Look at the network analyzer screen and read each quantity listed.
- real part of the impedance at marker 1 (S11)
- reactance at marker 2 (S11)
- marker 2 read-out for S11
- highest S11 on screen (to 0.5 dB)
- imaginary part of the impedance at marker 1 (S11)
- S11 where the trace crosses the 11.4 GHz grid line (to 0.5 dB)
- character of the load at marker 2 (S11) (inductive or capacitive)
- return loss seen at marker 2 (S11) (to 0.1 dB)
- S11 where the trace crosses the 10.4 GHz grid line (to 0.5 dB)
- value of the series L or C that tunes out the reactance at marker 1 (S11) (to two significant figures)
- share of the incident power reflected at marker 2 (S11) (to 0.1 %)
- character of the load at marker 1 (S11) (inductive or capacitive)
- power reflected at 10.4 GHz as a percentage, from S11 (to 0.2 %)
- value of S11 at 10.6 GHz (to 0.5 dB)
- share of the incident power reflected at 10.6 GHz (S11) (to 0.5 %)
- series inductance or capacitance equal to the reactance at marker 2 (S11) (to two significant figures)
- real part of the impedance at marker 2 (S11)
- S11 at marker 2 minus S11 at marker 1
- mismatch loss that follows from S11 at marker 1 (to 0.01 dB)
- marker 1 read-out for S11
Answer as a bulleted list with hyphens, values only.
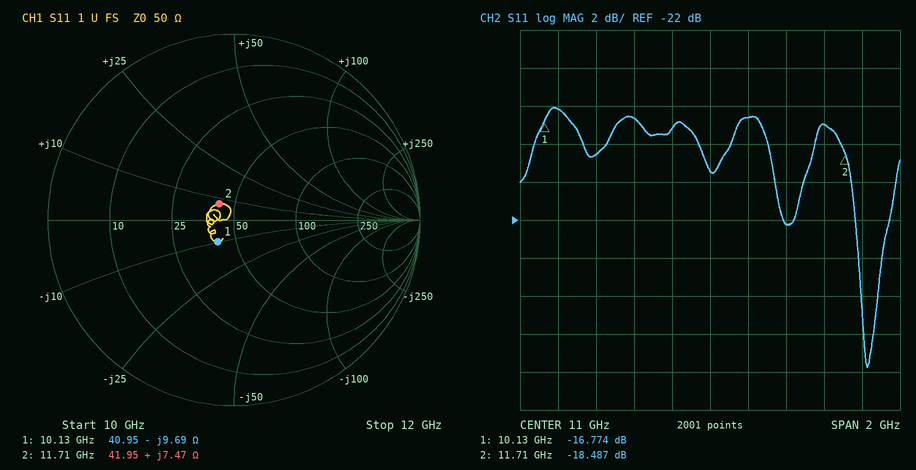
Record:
- 40.95 Ω
- +7.47 Ω
- -18.487 dB
- -16.0 dB
- -9.69 Ω
- -22.0 dB
- inductive
- 18.5 dB
- -18.5 dB
- 150 pH
- 1.4 %
- capacitive
- 1.4 %
- -16.5 dB
- 2.0 %
- 100 pH
- 41.95 Ω
- -1.713 dB
- 0.09 dB
- -16.774 dB
